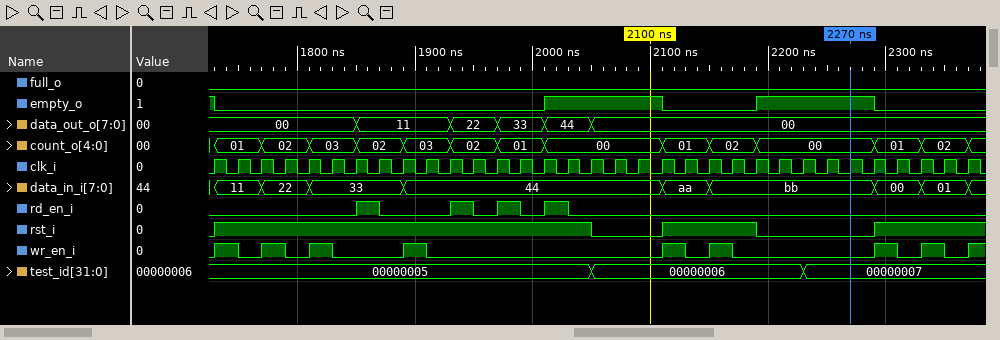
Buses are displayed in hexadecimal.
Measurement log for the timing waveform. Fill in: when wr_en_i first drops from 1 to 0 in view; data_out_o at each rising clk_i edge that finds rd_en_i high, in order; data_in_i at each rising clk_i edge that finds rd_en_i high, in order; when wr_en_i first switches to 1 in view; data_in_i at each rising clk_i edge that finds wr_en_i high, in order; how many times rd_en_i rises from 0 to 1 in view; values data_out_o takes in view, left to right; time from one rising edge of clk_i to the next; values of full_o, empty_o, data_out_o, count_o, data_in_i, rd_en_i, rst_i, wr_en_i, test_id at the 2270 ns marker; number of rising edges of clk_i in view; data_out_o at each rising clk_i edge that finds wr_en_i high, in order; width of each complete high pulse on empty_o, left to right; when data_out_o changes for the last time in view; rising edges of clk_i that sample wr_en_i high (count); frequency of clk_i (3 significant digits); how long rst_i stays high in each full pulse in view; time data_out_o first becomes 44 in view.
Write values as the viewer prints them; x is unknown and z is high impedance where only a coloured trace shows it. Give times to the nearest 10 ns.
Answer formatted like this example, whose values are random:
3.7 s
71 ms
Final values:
1750 ns
11, 22, 33, 44
33, 44, 44, 44
1730 ns
11, 22, 33, 44, aa, bb, 00, 01
4
00, 11, 22, 33, 44, 00
20 ns
full_o=0, empty_o=1, data_out_o=00, count_o=00, data_in_i=bb, rd_en_i=0, rst_i=0, wr_en_i=0, test_id=00000007
33
00, 00, 00, 11, 00, 00, 00, 00
100 ns, 100 ns
2050 ns
8
50.0 MHz
320 ns, 80 ns
2010 ns
